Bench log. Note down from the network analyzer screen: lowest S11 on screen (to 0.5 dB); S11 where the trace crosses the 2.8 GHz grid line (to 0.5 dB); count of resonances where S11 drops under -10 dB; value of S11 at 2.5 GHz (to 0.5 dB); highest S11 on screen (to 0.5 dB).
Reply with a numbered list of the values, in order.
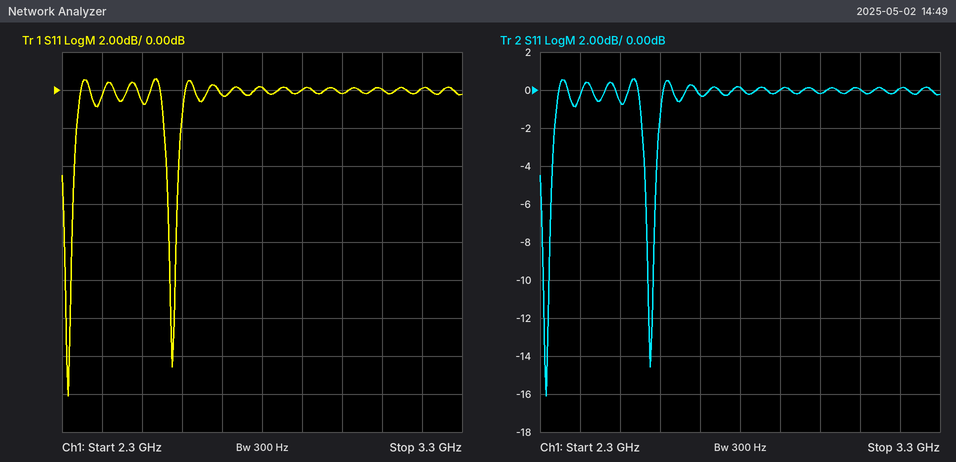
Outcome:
1. -16.0 dB
2. 0.0 dB
3. 2
4. -0.5 dB
5. 0.5 dB
